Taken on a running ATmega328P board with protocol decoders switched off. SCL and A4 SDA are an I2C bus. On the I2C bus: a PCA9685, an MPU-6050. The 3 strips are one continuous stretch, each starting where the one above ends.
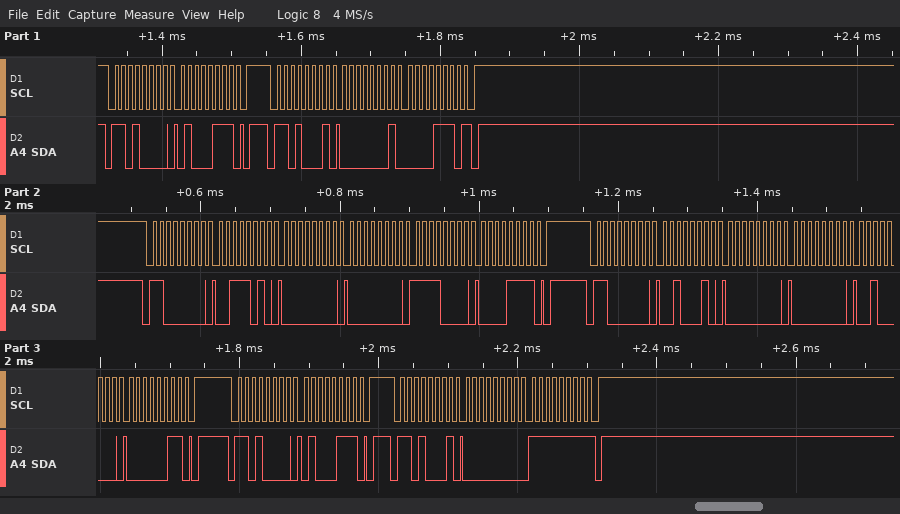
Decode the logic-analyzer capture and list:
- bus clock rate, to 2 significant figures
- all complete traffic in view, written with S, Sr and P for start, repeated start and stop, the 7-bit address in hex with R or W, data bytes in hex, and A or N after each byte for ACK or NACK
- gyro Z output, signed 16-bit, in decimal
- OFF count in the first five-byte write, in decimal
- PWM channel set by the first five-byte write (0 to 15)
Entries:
100 kHz
S 68W A 47 A P S 68R A 01 A 0E N P S 60W A 3A A 00 A 00 A F0 A 0F A P S 60W A 22 A 00 A 00 A 20 A 03 A P S 68W A 47 A P S 68R A 00 A FF N P
270
4080
13
